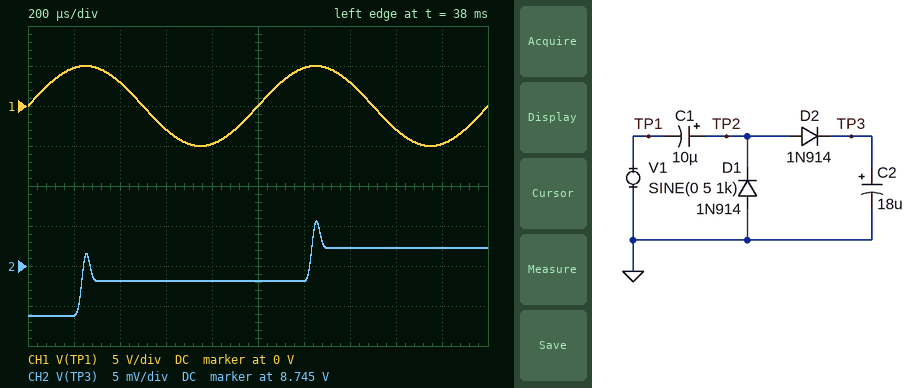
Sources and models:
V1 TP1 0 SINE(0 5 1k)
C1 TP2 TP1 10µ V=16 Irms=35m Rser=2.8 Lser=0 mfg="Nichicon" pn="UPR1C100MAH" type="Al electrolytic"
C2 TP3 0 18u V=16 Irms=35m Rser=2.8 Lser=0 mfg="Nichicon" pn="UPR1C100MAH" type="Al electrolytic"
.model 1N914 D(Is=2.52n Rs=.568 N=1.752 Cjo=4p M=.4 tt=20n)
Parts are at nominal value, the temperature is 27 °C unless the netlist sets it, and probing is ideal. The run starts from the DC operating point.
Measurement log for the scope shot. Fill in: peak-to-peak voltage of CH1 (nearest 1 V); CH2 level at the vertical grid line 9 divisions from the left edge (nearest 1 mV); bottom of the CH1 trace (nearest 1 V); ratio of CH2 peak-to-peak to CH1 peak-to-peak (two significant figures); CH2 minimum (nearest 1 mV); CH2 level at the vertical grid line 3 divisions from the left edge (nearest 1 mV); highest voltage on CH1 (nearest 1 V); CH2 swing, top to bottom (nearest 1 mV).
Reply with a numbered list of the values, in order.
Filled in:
1. 10 V
2. 8.747 V
3. -5 V
4. 0.0012
5. 8.739 V
6. 8.743 V
7. 5 V
8. 12 mV
